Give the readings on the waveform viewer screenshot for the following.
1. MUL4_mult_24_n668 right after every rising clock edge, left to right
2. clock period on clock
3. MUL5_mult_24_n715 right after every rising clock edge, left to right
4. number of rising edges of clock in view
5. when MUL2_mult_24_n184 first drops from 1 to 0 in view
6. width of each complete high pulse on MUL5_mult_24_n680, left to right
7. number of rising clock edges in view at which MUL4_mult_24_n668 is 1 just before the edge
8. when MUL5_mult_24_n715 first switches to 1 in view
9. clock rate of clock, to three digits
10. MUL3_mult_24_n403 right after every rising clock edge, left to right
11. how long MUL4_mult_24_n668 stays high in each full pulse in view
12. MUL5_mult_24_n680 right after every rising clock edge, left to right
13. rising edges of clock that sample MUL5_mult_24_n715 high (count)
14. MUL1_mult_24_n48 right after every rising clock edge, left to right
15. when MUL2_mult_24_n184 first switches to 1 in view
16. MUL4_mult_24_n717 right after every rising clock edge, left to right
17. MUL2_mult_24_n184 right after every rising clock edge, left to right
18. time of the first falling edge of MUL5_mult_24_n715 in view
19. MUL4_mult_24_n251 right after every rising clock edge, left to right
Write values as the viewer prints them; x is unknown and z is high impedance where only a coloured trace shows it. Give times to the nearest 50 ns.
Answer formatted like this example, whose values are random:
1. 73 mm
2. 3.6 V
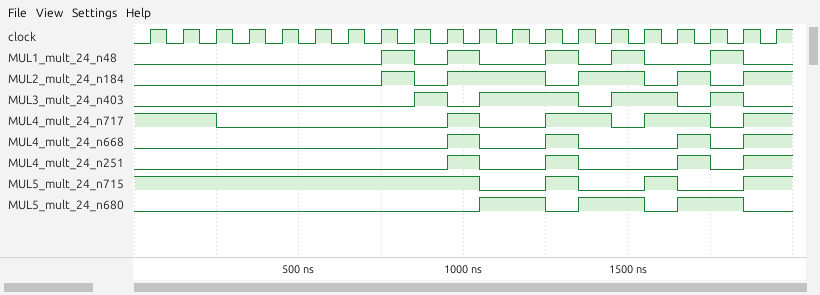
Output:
1. 0 0 0 0 0 0 0 0 0 1 0 0 1 0 0 0 1 0 1 1
2. 100 ns
3. 1 1 1 1 1 1 1 1 1 1 0 0 1 0 0 1 0 0 1 1
4. 20
5. 850 ns
6. 200 ns, 200 ns, 200 ns
7. 4
8. 1250 ns
9. 10.0 MHz
10. 0 0 0 0 0 0 0 0 1 0 1 1 1 0 1 1 0 1 0 0
11. 100 ns, 100 ns, 100 ns
12. 0 0 0 0 0 0 0 0 0 0 1 1 0 1 1 0 1 1 0 0
13. 14
14. 0 0 0 0 0 0 0 1 0 1 0 0 1 0 1 0 0 1 0 0
15. 750 ns
16. 1 1 0 0 0 0 0 0 0 1 0 0 1 1 0 1 1 0 1 1
17. 0 0 0 0 0 0 0 1 0 1 1 1 0 1 1 0 1 0 1 1
18. 1050 ns
19. 0 0 0 0 0 0 0 0 0 1 0 0 1 0 0 0 1 0 1 1
